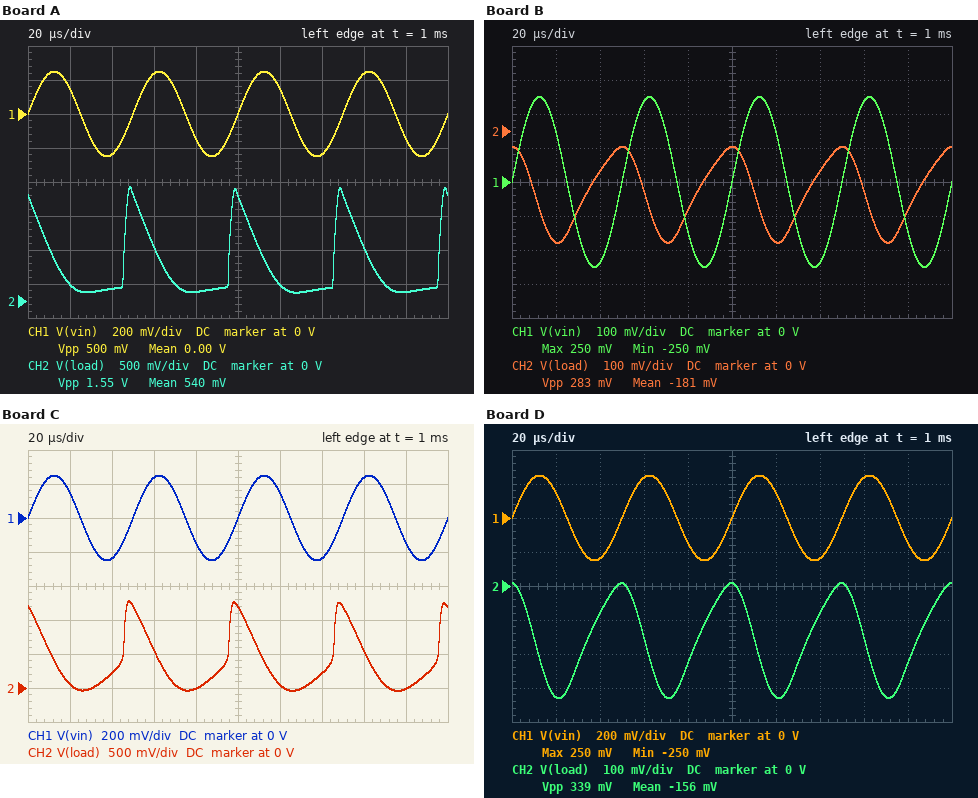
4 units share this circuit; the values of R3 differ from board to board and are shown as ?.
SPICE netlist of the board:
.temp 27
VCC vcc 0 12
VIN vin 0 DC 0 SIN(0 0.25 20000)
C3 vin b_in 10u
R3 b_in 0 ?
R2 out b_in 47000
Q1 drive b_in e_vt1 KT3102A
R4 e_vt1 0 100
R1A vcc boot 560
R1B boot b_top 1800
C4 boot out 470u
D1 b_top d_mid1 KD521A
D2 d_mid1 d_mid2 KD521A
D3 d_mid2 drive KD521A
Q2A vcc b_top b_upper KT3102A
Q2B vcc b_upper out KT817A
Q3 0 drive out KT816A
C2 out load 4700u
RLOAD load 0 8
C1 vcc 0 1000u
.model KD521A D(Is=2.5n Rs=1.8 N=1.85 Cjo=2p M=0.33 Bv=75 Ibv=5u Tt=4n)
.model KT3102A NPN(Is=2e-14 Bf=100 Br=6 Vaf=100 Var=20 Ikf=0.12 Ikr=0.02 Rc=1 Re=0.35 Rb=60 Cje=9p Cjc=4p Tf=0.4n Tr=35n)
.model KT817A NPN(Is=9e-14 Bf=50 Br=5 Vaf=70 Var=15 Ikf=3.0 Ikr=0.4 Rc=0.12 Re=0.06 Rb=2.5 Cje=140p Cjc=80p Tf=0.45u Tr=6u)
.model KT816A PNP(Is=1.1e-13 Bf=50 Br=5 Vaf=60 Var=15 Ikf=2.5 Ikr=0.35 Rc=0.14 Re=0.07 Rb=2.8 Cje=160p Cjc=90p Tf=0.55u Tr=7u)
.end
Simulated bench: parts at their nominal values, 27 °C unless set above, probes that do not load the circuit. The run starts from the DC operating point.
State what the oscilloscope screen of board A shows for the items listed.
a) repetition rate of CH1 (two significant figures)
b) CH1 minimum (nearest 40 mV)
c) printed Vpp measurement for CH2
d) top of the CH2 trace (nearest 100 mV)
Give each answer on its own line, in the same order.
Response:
20 kHz
-240 mV
1.55 V
1.7 V
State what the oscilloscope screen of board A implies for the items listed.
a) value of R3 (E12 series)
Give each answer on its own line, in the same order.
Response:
4.7 kΩ
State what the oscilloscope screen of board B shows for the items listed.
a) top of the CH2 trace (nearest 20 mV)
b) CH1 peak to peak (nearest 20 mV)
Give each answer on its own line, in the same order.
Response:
-40 mV
500 mV
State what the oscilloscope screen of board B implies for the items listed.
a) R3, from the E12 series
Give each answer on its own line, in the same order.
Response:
3.3 kΩ
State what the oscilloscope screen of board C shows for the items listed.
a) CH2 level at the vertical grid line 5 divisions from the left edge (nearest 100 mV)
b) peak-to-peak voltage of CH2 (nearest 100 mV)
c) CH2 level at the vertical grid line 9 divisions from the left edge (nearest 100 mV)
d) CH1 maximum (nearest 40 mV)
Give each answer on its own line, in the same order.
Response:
1.2 V
1.3 V
0 V
240 mV
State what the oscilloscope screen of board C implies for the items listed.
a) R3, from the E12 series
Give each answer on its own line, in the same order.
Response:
15 kΩ
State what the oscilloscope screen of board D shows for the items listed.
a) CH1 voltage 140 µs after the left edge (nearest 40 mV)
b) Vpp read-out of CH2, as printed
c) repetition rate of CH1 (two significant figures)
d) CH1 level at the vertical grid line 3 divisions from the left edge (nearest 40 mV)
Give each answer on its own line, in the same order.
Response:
-240 mV
339 mV
20 kHz
240 mV
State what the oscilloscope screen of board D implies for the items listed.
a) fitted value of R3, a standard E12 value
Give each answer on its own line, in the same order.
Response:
3.9 kΩ
